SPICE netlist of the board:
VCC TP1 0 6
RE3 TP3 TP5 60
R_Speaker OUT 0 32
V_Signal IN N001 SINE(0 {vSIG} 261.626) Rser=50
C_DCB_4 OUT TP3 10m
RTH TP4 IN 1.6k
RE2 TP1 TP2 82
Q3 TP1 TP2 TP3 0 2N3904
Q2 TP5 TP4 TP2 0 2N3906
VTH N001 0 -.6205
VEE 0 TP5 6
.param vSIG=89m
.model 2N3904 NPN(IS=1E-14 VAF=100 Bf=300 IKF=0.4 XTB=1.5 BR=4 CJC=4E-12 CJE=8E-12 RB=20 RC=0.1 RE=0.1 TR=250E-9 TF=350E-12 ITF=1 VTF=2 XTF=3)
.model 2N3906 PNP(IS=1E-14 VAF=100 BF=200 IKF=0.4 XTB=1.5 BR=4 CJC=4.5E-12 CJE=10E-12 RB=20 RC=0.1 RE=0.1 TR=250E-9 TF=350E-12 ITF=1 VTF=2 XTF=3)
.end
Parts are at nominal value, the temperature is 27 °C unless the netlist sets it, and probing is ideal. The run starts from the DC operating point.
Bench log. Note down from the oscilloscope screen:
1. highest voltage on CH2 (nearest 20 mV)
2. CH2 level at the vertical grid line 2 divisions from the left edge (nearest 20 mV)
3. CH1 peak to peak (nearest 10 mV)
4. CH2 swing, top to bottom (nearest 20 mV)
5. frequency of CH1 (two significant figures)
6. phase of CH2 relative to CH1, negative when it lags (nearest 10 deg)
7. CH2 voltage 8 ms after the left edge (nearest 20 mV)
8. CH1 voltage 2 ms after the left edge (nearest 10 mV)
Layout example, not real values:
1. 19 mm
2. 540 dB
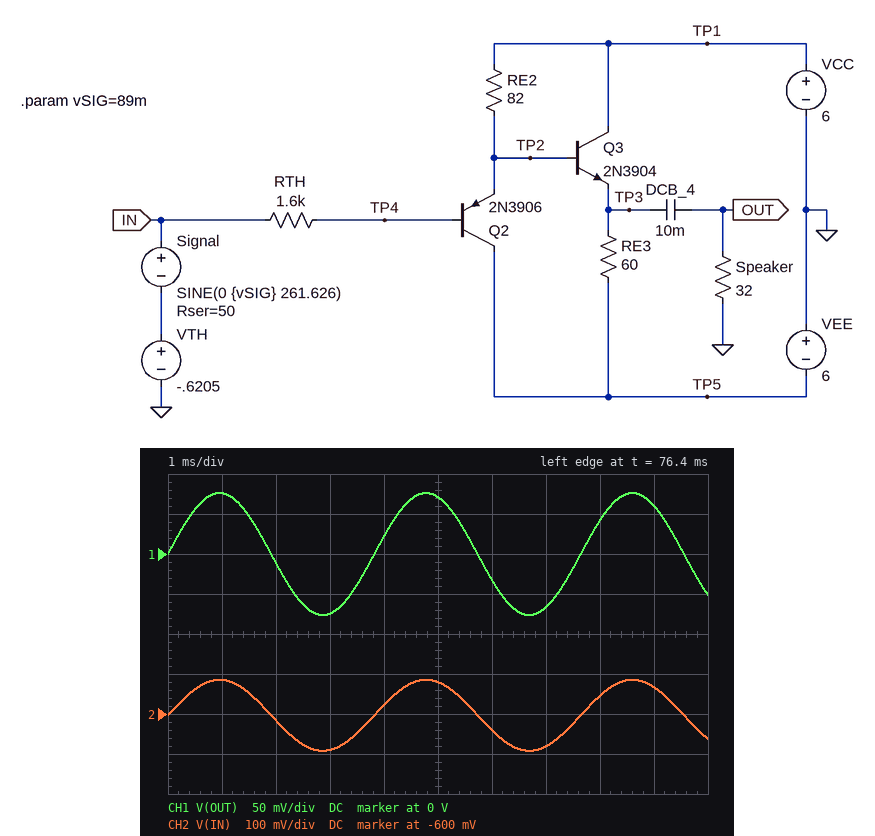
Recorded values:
1. -520 mV
2. -620 mV
3. 150 mV
4. 180 mV
5. 260 Hz
6. 0 deg
7. -560 mV
8. -10 mV
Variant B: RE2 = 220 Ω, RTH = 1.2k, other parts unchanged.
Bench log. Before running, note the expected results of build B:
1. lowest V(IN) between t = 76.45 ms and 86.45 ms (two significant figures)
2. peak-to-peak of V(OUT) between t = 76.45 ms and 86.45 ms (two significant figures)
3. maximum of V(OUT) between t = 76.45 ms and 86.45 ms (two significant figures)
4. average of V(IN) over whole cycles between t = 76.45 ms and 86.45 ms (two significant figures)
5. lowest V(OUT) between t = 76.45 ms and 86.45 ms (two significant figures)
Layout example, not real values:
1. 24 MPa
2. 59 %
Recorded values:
1. -700 mV
2. 170 mV
3. 83 mV
4. -610 mV
5. -84 mV
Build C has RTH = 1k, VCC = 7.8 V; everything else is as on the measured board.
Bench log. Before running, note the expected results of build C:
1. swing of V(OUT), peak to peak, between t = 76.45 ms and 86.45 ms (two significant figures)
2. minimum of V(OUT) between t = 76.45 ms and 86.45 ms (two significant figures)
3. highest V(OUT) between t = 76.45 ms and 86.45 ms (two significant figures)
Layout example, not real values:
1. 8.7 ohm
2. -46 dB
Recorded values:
1. 160 mV
2. -79 mV
3. 79 mV
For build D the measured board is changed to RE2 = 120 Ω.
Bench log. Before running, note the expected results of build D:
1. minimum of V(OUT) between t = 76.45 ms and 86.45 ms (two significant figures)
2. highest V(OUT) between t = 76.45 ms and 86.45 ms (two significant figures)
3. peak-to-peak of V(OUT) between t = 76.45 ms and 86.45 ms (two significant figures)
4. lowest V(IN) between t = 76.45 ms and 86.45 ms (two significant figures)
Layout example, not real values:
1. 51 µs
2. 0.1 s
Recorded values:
1. -80 mV
2. 79 mV
3. 160 mV
4. -700 mV
